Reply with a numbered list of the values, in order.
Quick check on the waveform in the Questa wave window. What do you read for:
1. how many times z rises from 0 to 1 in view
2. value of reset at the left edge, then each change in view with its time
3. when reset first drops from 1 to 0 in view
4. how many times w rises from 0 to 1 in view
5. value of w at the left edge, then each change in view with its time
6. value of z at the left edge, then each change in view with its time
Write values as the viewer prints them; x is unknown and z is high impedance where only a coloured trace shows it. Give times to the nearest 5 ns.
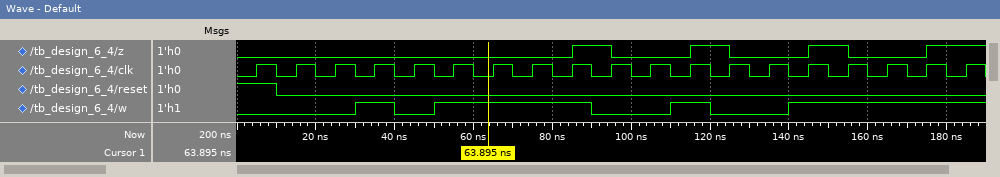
1. 4
2. 1, 0 at 10 ns
3. 10 ns
4. 4
5. 0, 1 at 30 ns, 0 at 40 ns, 1 at 50 ns, 0 at 90 ns, 1 at 110 ns, 0 at 120 ns, 1 at 140 ns
6. 0, 1 at 85 ns, 0 at 95 ns, 1 at 115 ns, 0 at 125 ns, 1 at 145 ns, 0 at 155 ns, 1 at 175 ns
